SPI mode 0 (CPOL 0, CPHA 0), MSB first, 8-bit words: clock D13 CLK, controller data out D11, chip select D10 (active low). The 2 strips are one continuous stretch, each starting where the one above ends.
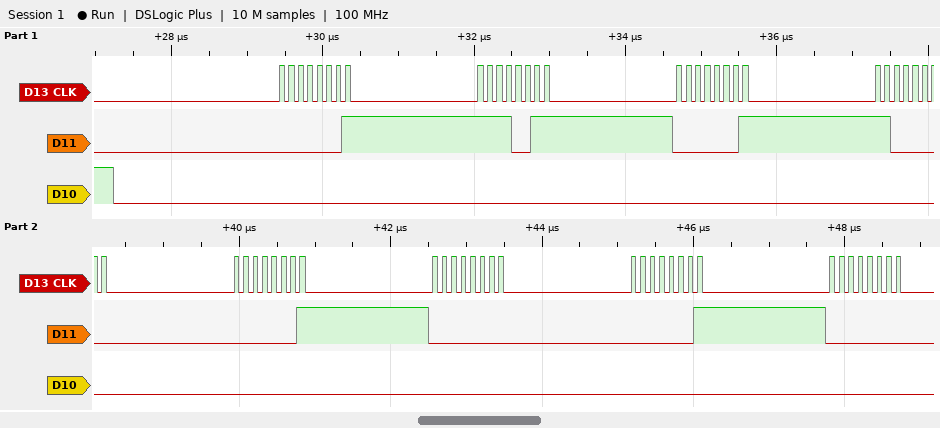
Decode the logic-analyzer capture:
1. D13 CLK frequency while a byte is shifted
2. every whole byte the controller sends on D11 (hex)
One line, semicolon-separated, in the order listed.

8 MHz; 0x01 0xF3 0x01 0xC0 0x01 0x00 0x01 0x00
